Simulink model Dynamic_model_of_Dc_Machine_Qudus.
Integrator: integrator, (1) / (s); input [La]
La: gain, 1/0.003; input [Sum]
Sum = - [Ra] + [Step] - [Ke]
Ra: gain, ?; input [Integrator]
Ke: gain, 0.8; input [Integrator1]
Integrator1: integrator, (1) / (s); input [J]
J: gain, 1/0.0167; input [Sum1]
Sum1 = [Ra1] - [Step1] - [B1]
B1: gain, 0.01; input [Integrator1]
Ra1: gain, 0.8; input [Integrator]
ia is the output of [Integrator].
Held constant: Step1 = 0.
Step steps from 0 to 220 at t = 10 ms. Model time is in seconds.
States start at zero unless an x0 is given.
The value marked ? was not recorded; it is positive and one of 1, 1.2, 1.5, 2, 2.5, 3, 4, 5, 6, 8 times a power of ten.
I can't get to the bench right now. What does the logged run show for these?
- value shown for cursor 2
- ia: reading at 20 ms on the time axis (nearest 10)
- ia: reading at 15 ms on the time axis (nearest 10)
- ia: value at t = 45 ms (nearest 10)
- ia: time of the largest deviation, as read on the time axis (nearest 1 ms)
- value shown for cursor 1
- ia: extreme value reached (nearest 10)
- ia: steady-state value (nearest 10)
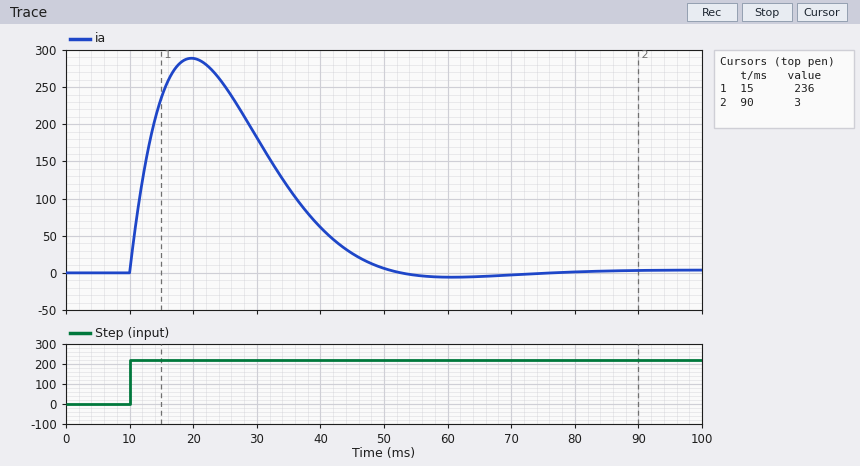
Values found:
3
290
240
30
20 ms
236
290
0
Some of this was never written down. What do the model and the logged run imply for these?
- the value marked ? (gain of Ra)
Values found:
0.5
